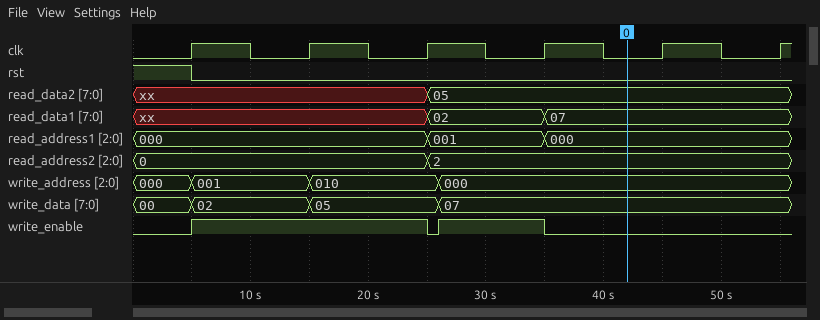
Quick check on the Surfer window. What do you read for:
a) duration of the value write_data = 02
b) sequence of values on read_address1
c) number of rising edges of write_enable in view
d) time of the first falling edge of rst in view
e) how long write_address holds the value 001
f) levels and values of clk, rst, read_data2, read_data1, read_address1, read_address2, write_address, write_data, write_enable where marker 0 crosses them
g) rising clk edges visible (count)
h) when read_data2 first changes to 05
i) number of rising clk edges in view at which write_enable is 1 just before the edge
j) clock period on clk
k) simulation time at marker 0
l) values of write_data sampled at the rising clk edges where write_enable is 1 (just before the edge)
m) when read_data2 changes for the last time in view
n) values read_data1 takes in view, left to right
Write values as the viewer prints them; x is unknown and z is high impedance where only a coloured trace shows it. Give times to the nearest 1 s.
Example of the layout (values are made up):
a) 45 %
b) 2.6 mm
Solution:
a) 10 s
b) 000, 001, 000
c) 2
d) 5 s
e) 10 s
f) clk=0, rst=0, read_data2=05, read_data1=07, read_address1=000, read_address2=2, write_address=000, write_data=07, write_enable=0
g) 6
h) 25 s
i) 3
j) 10 s
k) 42 s
l) 02, 05, 07
m) 25 s
n) xx, 02, 07
